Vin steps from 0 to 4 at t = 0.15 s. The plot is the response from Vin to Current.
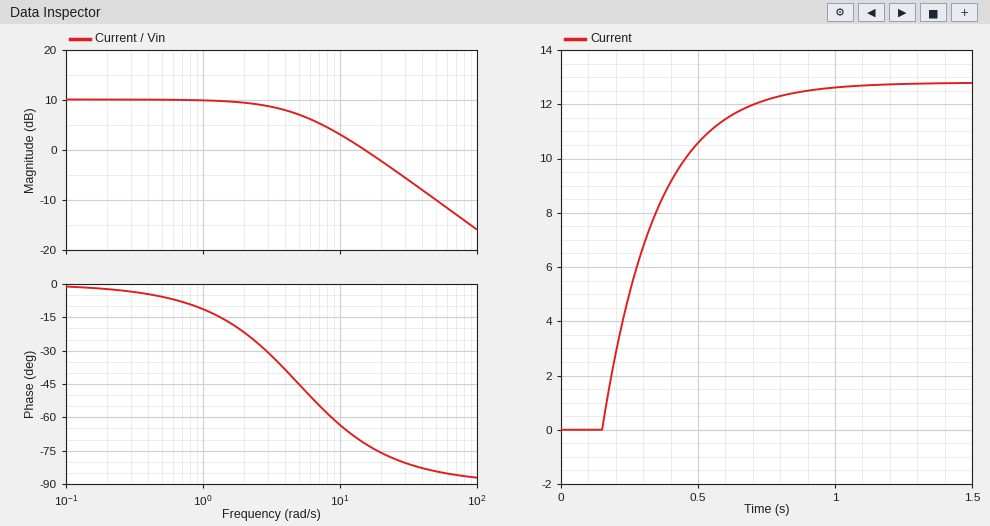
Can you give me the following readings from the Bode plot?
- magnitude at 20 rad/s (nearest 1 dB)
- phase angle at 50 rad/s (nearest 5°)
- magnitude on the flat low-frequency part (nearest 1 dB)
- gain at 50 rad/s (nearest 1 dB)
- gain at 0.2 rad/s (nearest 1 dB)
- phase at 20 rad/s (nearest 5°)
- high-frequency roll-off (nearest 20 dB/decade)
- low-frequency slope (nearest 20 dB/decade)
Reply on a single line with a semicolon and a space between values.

-2 dB; -85°; 10 dB; -10 dB; 10 dB; -75°; -20 dB/decade; 0 dB/decade
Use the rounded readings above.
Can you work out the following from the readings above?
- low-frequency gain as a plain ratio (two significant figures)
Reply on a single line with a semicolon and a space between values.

3.2
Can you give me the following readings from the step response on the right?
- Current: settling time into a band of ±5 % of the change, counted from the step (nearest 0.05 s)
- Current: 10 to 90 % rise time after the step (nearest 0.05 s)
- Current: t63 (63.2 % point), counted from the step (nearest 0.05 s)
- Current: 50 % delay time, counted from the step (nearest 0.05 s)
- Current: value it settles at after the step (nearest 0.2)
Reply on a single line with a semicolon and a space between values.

0.60 s; 0.45 s; 0.20 s; 0.15 s; 12.8
